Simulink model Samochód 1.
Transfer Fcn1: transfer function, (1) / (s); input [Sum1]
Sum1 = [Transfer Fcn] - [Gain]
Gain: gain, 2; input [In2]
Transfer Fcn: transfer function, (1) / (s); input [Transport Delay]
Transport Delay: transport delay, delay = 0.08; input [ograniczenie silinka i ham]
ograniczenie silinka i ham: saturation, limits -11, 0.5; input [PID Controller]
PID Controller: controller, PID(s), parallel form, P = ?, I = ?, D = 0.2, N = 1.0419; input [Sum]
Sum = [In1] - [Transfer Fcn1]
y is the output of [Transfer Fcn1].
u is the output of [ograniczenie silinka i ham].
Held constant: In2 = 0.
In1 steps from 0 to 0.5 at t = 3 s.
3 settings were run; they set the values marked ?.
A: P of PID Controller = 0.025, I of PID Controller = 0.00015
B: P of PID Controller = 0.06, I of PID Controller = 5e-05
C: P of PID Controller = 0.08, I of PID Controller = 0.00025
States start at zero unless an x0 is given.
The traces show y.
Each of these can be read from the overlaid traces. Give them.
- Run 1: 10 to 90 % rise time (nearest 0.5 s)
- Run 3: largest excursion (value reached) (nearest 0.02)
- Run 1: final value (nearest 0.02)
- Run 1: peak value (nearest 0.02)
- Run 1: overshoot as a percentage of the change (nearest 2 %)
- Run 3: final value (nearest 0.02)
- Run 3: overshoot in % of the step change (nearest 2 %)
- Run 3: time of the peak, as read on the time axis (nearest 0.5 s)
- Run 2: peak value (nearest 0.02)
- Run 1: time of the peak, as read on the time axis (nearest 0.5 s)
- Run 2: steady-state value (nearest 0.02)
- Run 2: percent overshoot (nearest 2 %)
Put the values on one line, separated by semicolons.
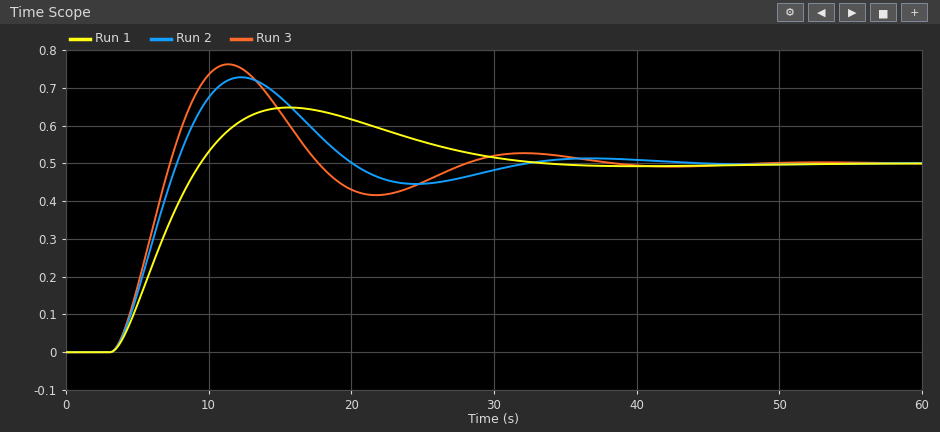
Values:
4.5 s; 0.76; 0.50; 0.64; 30 %; 0.50; 52 %; 11.5 s; 0.72; 15.5 s; 0.50; 46 %
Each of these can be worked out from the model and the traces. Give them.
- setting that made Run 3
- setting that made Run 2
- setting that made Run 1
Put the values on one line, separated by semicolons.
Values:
C; B; A
